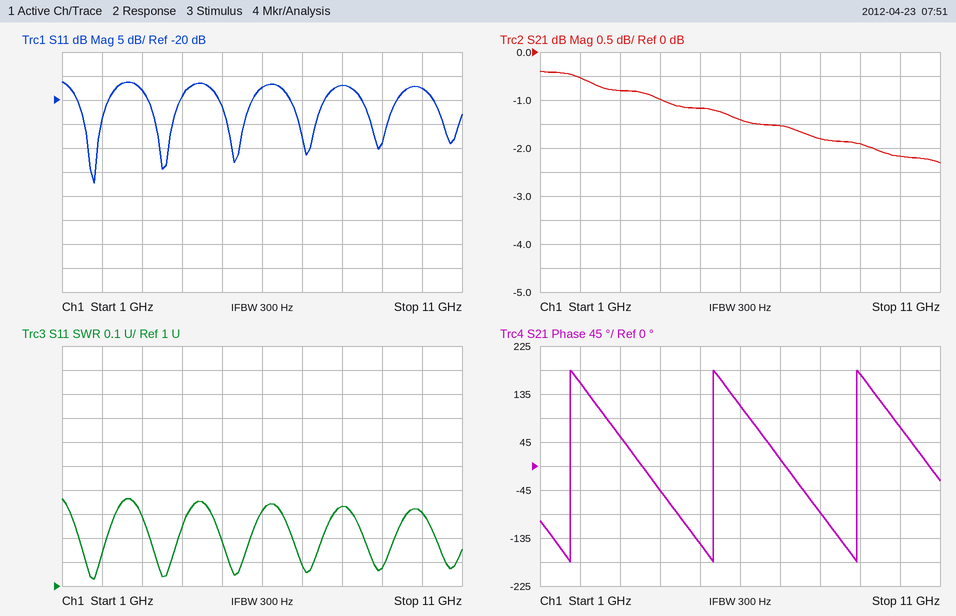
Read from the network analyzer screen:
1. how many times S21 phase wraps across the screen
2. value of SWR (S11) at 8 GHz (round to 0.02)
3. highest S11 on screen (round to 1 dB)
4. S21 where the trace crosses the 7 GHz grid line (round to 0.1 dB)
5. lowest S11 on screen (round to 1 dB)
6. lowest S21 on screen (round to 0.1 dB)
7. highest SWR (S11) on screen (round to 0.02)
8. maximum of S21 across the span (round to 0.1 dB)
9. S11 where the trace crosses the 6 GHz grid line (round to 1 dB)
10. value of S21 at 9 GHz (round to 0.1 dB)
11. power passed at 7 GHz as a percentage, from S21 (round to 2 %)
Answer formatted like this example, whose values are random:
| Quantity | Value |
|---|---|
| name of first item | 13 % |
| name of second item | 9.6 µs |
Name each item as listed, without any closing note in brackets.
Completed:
| Quantity | Value |
|---|---|
| how many times S21 phase wraps across the screen | 3 |
| value of SWR (S11) at 8 GHz | 1.34 |
| highest S11 on screen | -16 dB |
| S21 where the trace crosses the 7 GHz grid line | -1.5 dB |
| lowest S11 on screen | -37 dB |
| lowest S21 on screen | -2.3 dB |
| highest SWR (S11) on screen | 1.36 |
| maximum of S21 across the span | -0.4 dB |
| S11 where the trace crosses the 6 GHz grid line | -17 dB |
| value of S21 at 9 GHz | -1.9 dB |
| power passed at 7 GHz as a percentage, from S21 | 70 % |
